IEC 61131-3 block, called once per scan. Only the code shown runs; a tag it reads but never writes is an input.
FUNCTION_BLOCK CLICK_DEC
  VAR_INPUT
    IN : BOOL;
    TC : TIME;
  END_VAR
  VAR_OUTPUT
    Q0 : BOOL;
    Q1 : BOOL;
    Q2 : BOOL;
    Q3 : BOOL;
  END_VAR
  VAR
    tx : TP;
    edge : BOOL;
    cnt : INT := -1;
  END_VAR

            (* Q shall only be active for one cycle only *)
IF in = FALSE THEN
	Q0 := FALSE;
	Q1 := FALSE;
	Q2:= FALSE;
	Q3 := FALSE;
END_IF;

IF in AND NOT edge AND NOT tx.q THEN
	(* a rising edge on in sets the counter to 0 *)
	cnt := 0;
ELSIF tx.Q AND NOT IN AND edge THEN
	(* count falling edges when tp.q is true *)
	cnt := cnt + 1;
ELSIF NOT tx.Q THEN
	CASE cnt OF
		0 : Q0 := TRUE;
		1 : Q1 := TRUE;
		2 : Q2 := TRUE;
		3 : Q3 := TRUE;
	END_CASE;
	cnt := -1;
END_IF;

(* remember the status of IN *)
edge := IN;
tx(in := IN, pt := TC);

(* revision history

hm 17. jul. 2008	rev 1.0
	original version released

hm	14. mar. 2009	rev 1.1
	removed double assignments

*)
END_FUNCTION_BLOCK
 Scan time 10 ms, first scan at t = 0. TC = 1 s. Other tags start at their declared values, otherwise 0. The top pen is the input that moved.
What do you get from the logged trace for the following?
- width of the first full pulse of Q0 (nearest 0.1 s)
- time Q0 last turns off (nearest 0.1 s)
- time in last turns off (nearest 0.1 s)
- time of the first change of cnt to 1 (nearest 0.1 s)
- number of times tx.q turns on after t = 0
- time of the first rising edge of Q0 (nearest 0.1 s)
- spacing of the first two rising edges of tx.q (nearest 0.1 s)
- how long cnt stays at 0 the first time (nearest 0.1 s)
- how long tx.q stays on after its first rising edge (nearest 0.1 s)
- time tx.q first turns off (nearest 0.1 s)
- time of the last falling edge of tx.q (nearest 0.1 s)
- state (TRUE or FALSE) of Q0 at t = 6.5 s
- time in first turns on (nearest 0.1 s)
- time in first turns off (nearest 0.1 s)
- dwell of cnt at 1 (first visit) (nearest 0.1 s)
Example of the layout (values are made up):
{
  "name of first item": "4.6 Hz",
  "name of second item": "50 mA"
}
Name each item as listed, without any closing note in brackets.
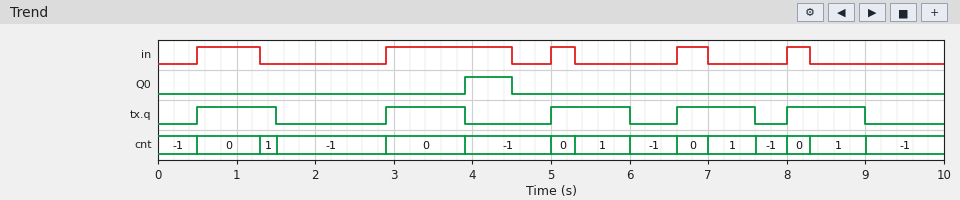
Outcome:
{
  "width of the first full pulse of Q0": "0.6 s",
  "time Q0 last turns off": "4.5 s",
  "time in last turns off": "8.3 s",
  "time of the first change of cnt to 1": "1.3 s",
  "number of times tx.q turns on after t = 0": "5",
  "time of the first rising edge of Q0": "3.9 s",
  "spacing of the first two rising edges of tx.q": "2.4 s",
  "how long cnt stays at 0 the first time": "0.8 s",
  "how long tx.q stays on after its first rising edge": "1.0 s",
  "time tx.q first turns off": "1.5 s",
  "time of the last falling edge of tx.q": "9.0 s",
  "state (TRUE or FALSE) of Q0 at t = 6.5 s": "FALSE",
  "time in first turns on": "0.5 s",
  "time in first turns off": "1.3 s",
  "dwell of cnt at 1 (first visit)": "0.2 s"
}
